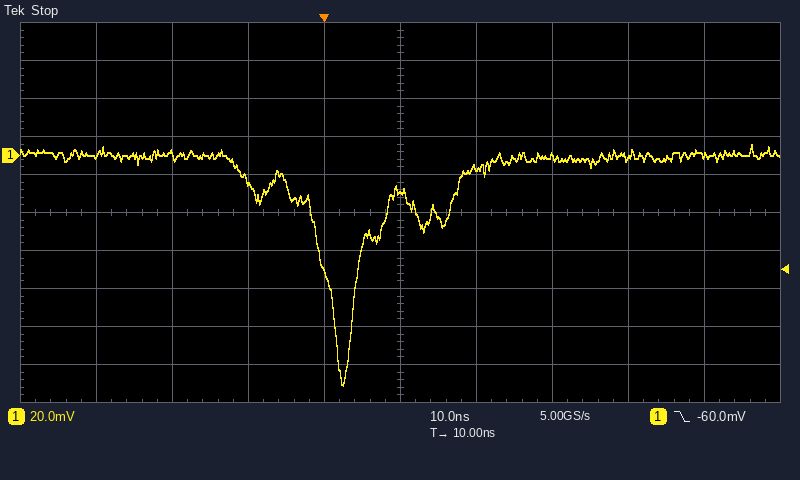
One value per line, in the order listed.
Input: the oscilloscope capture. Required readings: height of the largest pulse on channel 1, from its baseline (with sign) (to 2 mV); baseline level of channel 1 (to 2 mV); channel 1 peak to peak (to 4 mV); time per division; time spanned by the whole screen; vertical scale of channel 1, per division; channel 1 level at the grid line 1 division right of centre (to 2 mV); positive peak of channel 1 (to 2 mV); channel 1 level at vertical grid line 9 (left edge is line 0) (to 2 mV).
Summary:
-120 mV
0 mV
128 mV
10 ns
100 ns
20 mV
-6 mV
6 mV
0 mV
